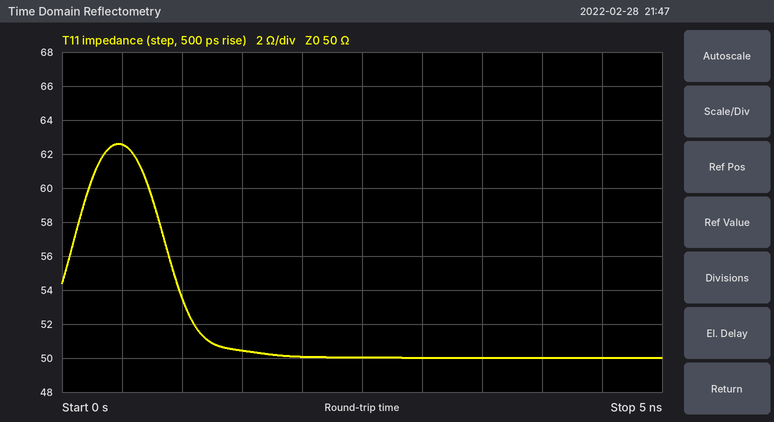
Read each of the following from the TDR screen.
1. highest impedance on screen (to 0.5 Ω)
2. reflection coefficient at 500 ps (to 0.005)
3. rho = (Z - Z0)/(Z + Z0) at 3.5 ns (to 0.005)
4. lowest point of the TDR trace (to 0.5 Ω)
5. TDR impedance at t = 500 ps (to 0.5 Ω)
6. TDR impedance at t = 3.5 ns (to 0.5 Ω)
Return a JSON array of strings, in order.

["62.5 Ω", "+0.110", "0.000", "50.0 Ω", "62.5 Ω", "50.0 Ω"]
